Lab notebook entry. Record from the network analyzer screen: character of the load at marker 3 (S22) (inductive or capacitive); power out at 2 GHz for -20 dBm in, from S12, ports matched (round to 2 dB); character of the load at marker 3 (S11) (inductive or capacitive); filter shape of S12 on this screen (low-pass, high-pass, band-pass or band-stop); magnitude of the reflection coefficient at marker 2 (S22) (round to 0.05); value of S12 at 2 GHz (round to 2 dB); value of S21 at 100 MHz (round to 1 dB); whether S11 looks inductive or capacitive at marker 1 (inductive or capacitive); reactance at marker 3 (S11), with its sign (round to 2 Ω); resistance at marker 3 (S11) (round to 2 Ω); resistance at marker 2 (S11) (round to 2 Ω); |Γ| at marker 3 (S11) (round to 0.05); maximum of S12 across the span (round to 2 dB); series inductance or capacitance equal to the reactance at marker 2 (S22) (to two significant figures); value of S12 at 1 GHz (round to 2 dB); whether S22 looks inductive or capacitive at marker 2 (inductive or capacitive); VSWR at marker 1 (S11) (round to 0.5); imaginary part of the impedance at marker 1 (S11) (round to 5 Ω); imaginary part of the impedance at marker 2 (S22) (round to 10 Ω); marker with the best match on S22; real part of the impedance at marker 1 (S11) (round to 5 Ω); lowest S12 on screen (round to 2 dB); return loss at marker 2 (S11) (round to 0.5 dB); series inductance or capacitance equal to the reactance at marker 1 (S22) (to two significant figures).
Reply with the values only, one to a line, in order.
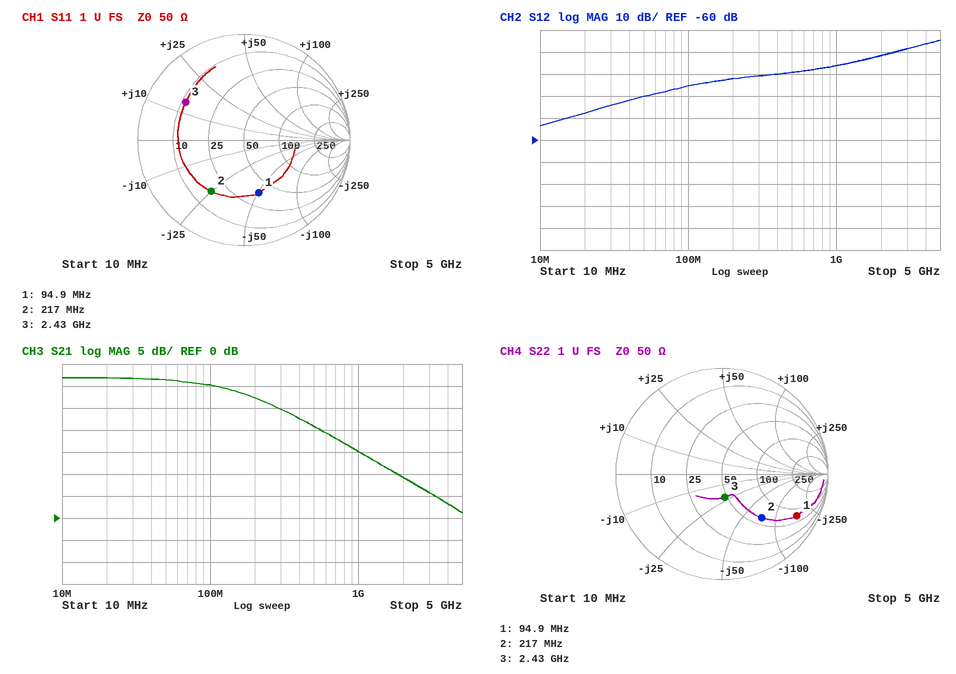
capacitive
-42 dBm
inductive
high-pass
0.55
-22 dB
30 dB
capacitive
+14 Ω
12 Ω
18 Ω
0.65
-14 dB
10 pF
-26 dB
capacitive
3.0
-50 Ω
-70 Ω
marker 3
35 Ω
-54 dB
5.0 dB
10 pF
